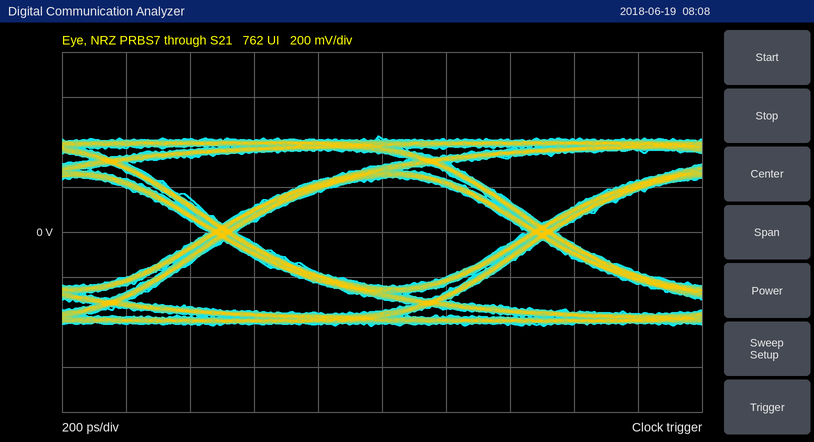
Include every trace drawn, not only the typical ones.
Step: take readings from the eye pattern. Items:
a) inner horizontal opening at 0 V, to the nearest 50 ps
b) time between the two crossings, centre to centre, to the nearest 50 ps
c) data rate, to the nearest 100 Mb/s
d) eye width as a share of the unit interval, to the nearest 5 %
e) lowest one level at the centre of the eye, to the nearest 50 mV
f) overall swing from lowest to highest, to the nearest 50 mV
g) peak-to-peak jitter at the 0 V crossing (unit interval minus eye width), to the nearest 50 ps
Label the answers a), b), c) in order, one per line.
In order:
a) 900 ps
b) 1.00 ns
c) 1.0 Gb/s
d) 90 %
e) 250 mV
f) 850 mV
g) 100 ps
